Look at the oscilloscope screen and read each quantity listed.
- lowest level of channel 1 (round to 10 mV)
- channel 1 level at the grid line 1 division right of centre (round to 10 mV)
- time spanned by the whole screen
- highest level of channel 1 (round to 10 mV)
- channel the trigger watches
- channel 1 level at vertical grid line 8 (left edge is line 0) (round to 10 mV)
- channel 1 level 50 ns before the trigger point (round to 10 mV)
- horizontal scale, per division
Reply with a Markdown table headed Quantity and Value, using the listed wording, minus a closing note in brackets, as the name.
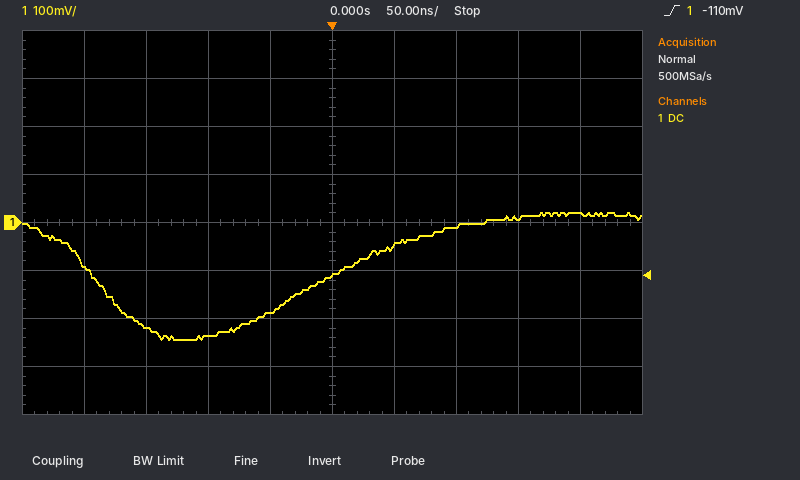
| Quantity | Value |
|---|---|
| lowest level of channel 1 | -240 mV |
| channel 1 level at the grid line 1 division right of centre | -50 mV |
| time spanned by the whole screen | 500 ns |
| highest level of channel 1 | 20 mV |
| channel the trigger watches | channel 1 |
| channel 1 level at vertical grid line 8 (left edge is line 0) | 10 mV |
| channel 1 level 50 ns before the trigger point | -190 mV |
| horizontal scale, per division | 50 ns |
